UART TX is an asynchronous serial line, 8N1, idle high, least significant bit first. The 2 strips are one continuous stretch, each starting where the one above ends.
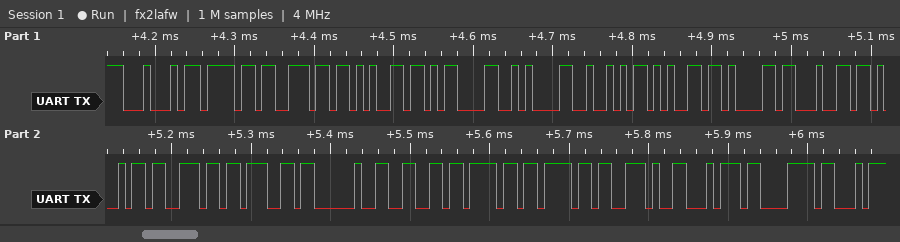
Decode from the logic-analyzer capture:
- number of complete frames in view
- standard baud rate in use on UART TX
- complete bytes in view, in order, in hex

20
115200 baud
0x44 0x6F 0x6E 0x65 0x0D 0x0A 0x52 0x65 0x61 0x64 0x69 0x6E 0x67 0x20 0x66 0x6F 0x6F 0x2E 0x74 0x78
